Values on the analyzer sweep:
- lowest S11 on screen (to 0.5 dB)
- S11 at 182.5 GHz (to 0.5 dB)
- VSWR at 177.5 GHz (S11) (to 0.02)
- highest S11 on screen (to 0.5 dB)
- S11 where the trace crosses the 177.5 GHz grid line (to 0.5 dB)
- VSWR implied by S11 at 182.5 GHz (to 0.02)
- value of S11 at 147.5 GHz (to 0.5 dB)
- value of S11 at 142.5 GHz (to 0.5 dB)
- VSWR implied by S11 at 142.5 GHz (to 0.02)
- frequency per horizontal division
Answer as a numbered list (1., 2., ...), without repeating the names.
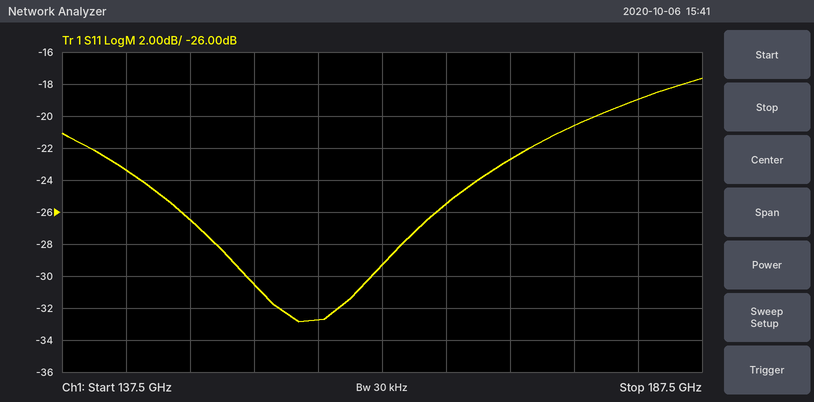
1. -33.0 dB
2. -19.0 dB
3. 1.20
4. -17.5 dB
5. -20.5 dB
6. 1.26
7. -26.5 dB
8. -23.5 dB
9. 1.14
10. 5 GHz
